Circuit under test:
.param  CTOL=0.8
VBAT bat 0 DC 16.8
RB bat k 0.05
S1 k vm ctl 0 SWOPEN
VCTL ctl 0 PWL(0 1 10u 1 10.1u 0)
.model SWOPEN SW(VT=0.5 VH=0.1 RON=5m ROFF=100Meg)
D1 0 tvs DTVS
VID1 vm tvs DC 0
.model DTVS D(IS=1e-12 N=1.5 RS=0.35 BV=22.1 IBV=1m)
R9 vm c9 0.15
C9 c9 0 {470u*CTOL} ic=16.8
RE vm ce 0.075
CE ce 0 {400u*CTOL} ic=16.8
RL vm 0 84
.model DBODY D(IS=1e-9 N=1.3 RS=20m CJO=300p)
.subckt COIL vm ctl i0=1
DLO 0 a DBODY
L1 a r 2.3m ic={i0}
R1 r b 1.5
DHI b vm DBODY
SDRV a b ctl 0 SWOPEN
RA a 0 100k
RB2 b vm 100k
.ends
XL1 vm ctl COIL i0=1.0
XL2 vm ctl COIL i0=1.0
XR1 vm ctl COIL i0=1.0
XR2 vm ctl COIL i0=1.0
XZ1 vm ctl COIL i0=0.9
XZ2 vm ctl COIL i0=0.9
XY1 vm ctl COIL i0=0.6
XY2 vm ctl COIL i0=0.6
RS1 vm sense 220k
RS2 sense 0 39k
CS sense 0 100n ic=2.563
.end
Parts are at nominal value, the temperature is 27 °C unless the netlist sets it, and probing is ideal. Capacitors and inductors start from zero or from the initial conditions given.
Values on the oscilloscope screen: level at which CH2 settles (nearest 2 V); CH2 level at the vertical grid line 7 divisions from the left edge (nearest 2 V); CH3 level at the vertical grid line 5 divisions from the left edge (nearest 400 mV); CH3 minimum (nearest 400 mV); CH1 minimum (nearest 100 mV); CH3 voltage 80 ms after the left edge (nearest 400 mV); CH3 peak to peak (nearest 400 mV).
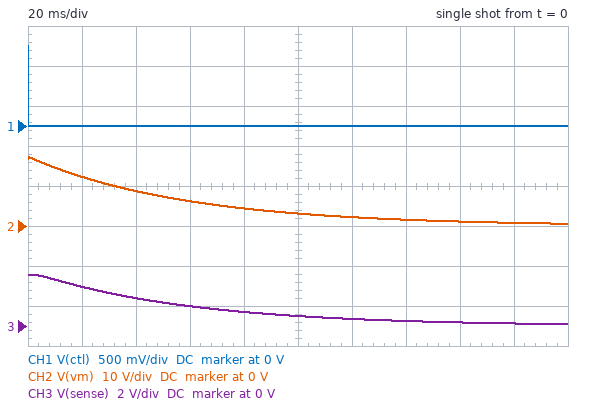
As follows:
0 V
2 V
400 mV
0 V
0 V
800 mV
2.4 V
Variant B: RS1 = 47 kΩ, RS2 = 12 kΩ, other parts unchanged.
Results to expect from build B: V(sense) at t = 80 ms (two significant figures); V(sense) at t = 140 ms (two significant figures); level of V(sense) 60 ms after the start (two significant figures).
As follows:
910 mV
320 mV
1.3 V
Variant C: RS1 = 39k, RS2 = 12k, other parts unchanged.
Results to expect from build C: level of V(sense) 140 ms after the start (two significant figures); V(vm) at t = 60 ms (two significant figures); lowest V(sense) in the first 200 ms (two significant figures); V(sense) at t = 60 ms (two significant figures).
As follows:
370 mV
6.2 V
130 mV
1.5 V
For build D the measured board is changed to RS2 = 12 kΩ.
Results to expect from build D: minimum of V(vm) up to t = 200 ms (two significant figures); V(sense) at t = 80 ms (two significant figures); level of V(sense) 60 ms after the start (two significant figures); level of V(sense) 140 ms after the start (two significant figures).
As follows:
560 mV
230 mV
330 mV
83 mV
